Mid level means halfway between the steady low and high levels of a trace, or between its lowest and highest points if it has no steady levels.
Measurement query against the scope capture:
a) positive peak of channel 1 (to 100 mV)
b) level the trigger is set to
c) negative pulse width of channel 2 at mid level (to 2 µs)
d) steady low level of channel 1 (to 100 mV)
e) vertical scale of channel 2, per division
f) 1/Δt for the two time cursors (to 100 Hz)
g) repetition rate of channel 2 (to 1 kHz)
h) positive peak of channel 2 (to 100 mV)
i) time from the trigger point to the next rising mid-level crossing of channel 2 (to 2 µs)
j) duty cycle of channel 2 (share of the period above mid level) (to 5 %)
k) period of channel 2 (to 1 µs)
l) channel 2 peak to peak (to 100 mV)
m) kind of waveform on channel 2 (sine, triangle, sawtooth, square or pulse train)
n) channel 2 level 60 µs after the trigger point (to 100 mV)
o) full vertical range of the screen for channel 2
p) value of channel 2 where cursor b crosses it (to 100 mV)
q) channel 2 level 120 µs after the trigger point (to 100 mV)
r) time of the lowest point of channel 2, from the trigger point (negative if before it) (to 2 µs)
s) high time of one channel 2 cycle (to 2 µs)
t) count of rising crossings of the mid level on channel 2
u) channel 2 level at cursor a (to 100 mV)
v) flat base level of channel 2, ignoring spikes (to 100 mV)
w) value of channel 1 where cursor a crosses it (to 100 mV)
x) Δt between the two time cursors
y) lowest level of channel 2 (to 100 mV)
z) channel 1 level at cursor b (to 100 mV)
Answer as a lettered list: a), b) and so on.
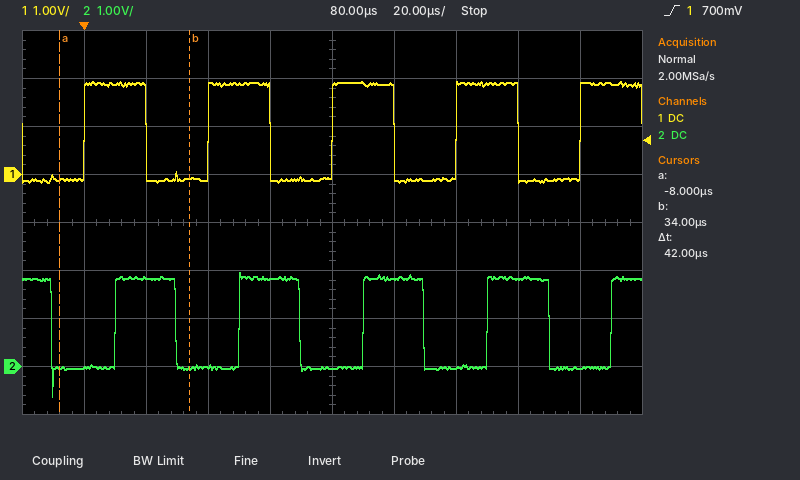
a) 1.9 V
b) 700 mV
c) 20 µs
d) -100 mV
e) 1 V
f) 23.8 kHz
g) 25 kHz
h) 2.0 V
i) 10 µs
j) 50 %
k) 40 µs
l) 2.6 V
m) square
n) 1.8 V
o) 8 V
p) 0.0 V
q) 0.0 V
r) -10 µs
s) 20 µs
t) 5
u) 0.0 V
v) 0.0 V
w) -100 mV
x) 42 µs
y) -600 mV
z) -100 mV
